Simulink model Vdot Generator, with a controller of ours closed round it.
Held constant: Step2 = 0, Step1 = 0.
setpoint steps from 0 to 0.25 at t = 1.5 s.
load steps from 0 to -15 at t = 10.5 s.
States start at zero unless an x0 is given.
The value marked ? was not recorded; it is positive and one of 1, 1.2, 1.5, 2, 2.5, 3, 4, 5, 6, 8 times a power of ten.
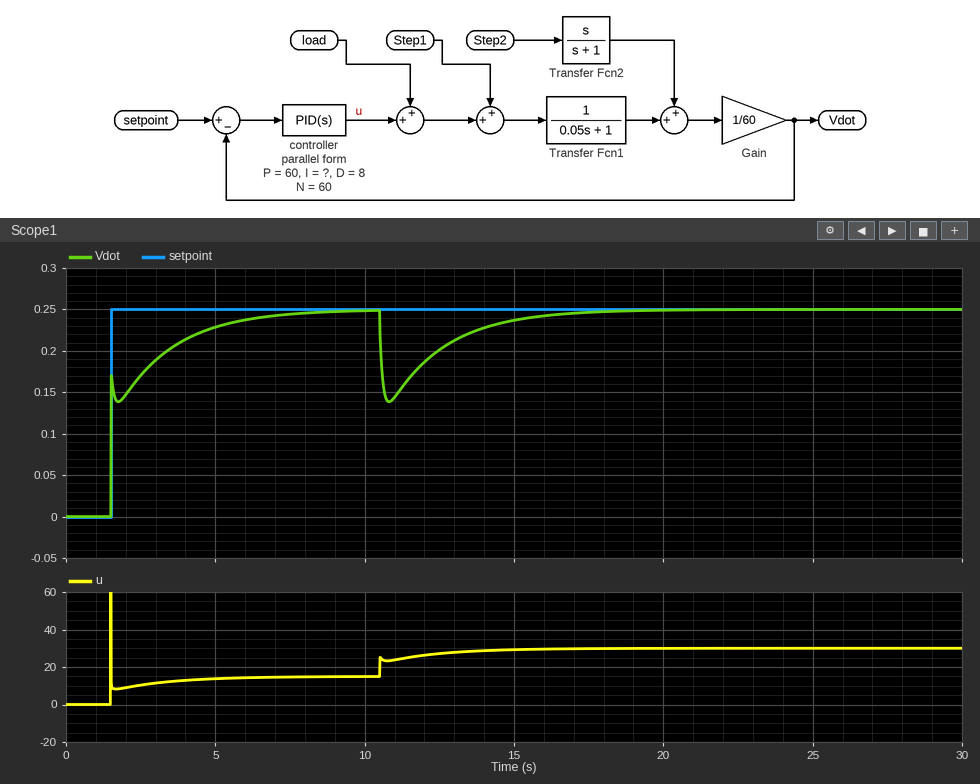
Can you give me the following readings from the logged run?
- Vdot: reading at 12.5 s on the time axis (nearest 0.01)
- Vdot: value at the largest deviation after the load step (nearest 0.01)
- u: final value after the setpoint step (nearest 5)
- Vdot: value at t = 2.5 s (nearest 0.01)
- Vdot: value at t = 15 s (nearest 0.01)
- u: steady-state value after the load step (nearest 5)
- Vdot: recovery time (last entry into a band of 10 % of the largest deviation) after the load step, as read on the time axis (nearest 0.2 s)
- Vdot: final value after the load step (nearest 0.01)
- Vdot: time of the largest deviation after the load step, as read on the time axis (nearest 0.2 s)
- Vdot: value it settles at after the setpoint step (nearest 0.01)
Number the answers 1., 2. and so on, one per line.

1. 0.20
2. 0.14
3. 15
4. 0.17
5. 0.24
6. 30
7. 15.4 s
8. 0.25
9. 10.8 s
10. 0.25
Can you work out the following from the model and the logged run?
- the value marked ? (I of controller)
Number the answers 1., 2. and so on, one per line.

1. 60
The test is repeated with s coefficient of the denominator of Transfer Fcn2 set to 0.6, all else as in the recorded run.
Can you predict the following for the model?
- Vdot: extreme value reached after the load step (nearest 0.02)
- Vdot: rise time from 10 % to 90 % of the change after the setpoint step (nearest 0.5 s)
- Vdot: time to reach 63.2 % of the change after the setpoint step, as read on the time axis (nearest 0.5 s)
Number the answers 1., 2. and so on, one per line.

1. 0.14
2. 3.0 s
3. 1.5 s
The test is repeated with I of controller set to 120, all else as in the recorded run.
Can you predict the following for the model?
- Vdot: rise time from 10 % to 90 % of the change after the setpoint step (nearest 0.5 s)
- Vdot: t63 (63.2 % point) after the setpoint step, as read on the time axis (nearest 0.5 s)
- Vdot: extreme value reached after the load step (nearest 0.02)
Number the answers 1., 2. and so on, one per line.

1. 1.5 s
2. 1.5 s
3. 0.14
